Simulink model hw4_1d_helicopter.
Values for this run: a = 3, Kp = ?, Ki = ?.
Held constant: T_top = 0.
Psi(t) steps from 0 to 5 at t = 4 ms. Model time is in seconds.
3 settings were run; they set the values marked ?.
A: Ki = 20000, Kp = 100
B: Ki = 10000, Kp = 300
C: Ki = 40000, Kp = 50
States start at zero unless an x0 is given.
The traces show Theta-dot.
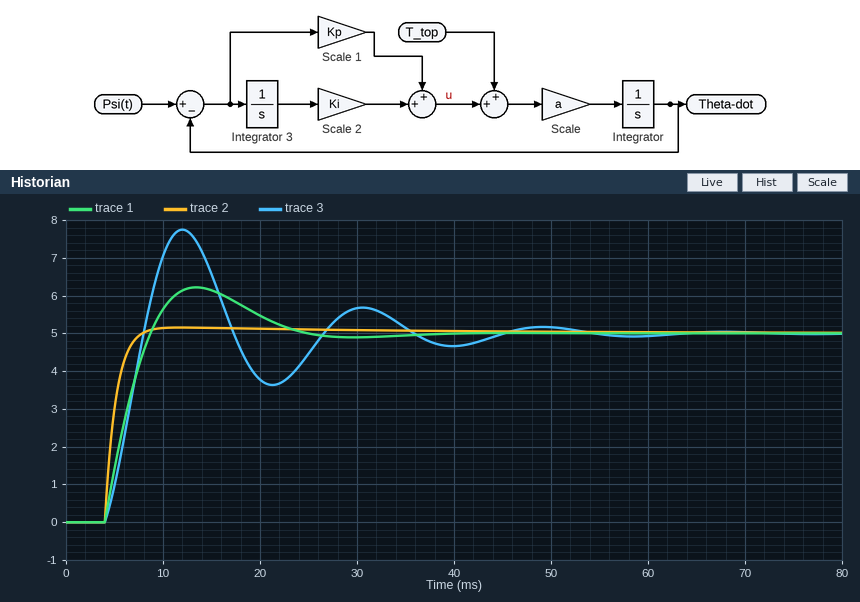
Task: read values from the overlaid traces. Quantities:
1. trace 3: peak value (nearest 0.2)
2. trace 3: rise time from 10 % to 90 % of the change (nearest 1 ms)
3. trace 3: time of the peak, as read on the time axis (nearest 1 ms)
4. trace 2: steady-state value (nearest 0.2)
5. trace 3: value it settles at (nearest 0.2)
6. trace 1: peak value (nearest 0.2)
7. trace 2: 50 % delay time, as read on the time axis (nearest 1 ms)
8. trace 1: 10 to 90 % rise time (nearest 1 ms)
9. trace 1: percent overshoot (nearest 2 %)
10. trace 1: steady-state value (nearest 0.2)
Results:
7.8
3 ms
12 ms
5.0
5.0
6.2
5 ms
4 ms
24 %
5.0
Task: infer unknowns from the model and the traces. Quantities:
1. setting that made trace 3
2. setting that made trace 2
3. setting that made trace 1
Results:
C
B
A
